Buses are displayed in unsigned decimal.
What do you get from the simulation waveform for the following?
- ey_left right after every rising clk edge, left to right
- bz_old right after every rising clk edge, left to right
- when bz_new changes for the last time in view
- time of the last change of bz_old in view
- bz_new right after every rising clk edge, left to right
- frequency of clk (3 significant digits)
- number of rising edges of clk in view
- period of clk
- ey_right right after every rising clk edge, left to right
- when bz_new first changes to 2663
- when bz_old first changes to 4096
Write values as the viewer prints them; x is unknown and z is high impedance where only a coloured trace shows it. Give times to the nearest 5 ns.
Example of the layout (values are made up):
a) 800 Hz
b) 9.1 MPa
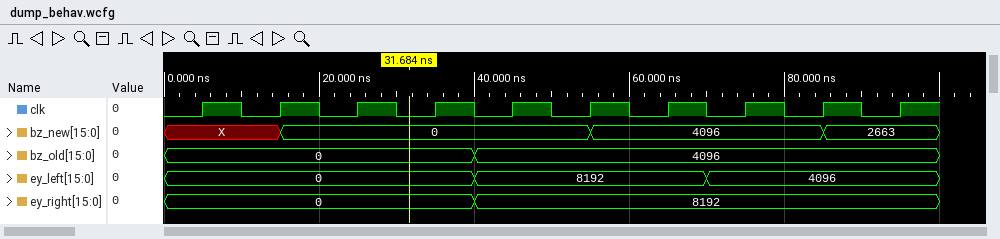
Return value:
a) 0, 0, 0, 0, 8192, 8192, 8192, 4096, 4096, 4096
b) 0, 0, 0, 0, 4096, 4096, 4096, 4096, 4096, 4096
c) 85 ns
d) 40 ns
e) X, 0, 0, 0, 0, 4096, 4096, 4096, 2663, 2663
f) 100 MHz
g) 10
h) 10 ns
i) 0, 0, 0, 0, 8192, 8192, 8192, 8192, 8192, 8192
j) 85 ns
k) 40 ns
